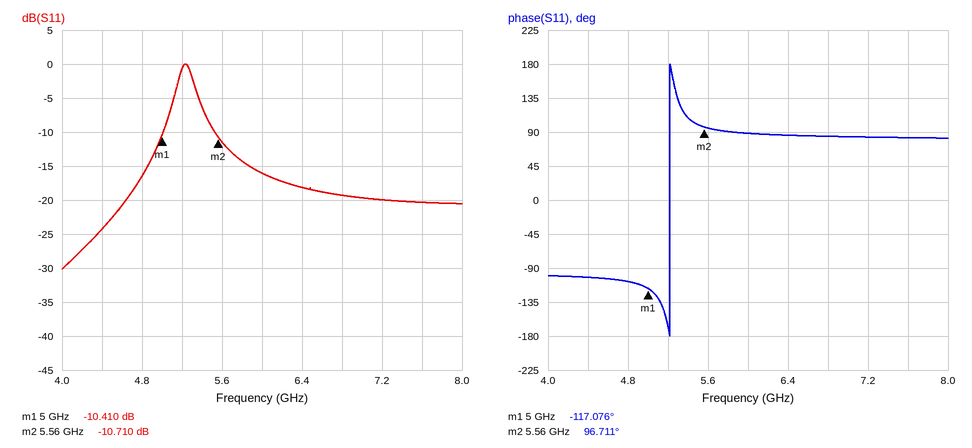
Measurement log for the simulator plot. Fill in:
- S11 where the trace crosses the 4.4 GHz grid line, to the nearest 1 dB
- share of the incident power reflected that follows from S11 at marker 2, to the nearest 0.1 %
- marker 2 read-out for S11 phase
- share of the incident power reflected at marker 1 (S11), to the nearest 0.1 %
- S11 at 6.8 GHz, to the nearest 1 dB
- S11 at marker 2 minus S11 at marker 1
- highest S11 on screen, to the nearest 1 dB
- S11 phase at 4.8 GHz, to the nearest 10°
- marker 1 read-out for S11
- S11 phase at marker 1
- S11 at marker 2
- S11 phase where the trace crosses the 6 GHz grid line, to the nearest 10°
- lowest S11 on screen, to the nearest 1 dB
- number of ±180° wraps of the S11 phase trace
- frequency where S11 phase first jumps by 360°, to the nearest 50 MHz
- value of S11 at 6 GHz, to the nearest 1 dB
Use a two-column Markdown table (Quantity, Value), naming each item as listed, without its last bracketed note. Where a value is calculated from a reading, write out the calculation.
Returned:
| Quantity | Value |
|---|---|
| S11 where the trace crosses the 4.4 GHz grid line, to the nearest 1 dB | -24 dB |
| share of the incident power reflected that follows from S11 at marker 2, to the nearest 0.1 % | 10^(-10.71/10) ≈ 8.5 % |
| marker 2 read-out for S11 phase | 96.711° |
| share of the incident power reflected at marker 1 (S11), to the nearest 0.1 % | 10^(-10.41/10) ≈ 9.1 % |
| S11 at 6.8 GHz, to the nearest 1 dB | -19 dB |
| S11 at marker 2 minus S11 at marker 1 | -10.71 − (-10.41) = -0.300 dB |
| highest S11 on screen, to the nearest 1 dB | 0 dB |
| S11 phase at 4.8 GHz, to the nearest 10° | -110° |
| marker 1 read-out for S11 | -10.410 dB |
| S11 phase at marker 1 | -117.076° |
| S11 at marker 2 | -10.710 dB |
| S11 phase where the trace crosses the 6 GHz grid line, to the nearest 10° | 90° |
| lowest S11 on screen, to the nearest 1 dB | -30 dB |
| number of ±180° wraps of the S11 phase trace | 1 |
| frequency where S11 phase first jumps by 360°, to the nearest 50 MHz | 5.20 GHz |
| value of S11 at 6 GHz, to the nearest 1 dB | -16 dB |
